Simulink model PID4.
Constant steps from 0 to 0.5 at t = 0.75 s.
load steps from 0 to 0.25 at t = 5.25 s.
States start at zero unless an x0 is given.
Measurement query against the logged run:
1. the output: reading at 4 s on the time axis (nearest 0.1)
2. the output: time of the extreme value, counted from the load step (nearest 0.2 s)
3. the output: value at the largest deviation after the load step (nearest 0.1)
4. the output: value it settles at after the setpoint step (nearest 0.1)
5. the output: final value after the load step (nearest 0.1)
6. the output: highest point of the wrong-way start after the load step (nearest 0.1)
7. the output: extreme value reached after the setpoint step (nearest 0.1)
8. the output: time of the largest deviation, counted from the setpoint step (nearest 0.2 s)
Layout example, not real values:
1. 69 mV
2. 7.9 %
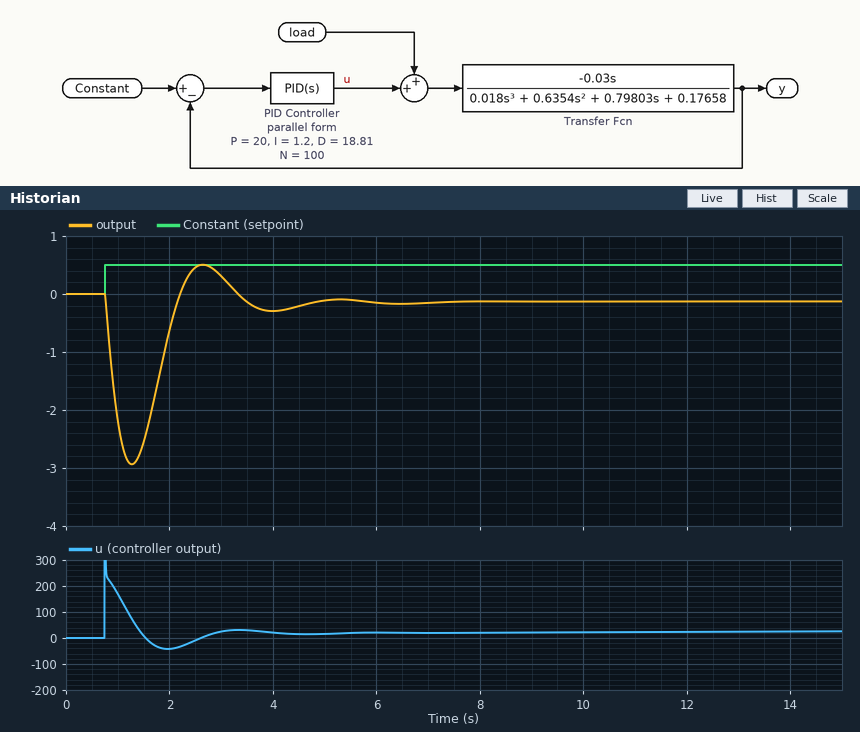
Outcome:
1. -0.3
2. 1.2 s
3. -0.2
4. -0.1
5. -0.1
6. -0.1
7. -2.9
8. 0.6 s
